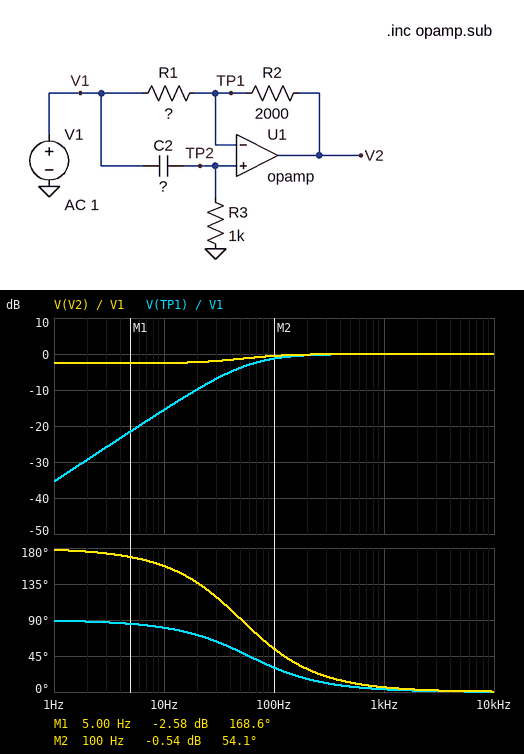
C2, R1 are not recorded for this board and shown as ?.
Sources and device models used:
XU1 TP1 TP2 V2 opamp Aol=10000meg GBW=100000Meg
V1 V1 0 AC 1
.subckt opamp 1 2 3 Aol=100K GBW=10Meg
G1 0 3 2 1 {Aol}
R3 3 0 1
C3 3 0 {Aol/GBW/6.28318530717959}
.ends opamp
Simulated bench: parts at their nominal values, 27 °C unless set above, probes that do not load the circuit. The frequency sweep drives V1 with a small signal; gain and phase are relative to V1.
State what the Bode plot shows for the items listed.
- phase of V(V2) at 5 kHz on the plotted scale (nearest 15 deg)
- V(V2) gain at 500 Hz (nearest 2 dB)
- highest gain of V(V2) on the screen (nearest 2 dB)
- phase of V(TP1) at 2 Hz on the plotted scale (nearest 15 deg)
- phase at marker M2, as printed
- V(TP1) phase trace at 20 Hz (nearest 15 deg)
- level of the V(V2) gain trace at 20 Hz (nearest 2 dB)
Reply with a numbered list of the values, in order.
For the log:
1. 0 deg
2. 0 dB
3. 0 dB
4. 90 deg
5. 54.1 deg
6. 75 deg
7. -2 dB
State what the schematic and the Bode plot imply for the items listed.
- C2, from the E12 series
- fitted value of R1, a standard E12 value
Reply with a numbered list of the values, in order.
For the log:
1. 2.7 µF
2. 2.7 kΩ
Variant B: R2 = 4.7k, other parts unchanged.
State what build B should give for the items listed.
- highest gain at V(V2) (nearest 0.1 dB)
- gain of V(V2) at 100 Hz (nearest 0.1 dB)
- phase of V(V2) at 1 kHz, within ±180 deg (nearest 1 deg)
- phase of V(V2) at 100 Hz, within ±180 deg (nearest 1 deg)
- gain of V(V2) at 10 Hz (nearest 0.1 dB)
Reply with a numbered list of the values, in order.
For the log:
1. 4.8 dB
2. 1.8 dB
3. 9 deg
4. 76 deg
5. 4.7 dB
